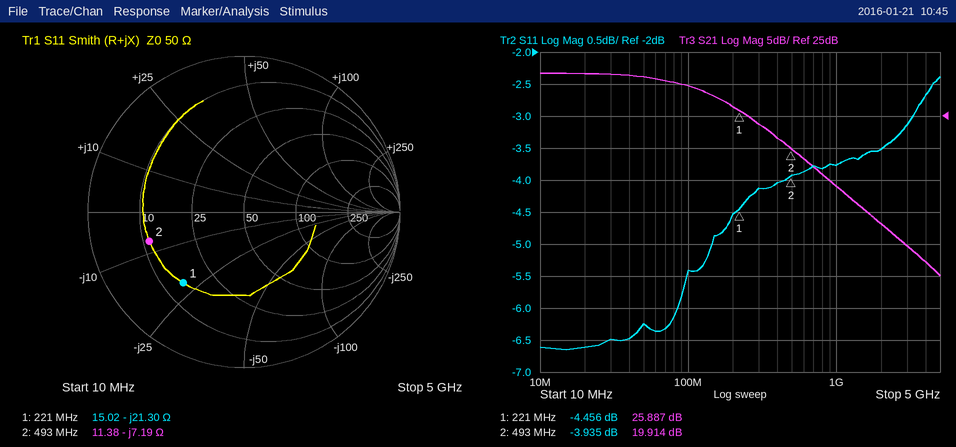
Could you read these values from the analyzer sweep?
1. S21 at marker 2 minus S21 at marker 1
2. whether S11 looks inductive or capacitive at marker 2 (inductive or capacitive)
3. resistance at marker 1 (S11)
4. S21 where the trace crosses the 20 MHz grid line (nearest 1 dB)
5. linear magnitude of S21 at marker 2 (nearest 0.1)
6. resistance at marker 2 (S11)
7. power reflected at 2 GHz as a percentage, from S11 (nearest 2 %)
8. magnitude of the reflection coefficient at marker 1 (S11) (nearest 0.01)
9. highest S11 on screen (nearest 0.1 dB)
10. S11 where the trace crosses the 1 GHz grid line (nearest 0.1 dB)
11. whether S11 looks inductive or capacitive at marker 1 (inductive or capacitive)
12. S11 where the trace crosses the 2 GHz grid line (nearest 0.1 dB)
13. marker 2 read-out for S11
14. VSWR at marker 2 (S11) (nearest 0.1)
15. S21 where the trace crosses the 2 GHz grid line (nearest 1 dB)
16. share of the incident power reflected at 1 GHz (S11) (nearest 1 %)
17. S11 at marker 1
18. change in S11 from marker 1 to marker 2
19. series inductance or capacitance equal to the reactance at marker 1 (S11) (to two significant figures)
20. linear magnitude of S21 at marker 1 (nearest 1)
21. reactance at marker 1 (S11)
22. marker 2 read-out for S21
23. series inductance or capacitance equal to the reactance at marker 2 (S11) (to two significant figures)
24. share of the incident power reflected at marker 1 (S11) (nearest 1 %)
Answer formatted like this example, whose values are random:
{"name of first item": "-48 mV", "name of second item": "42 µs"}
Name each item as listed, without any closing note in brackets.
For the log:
{"S21 at marker 2 minus S21 at marker 1": "-5.973 dB", "whether S11 looks inductive or capacitive at marker 2": "capacitive", "resistance at marker 1": "15.02 Ω", "S21 where the trace crosses the 20 MHz grid line": "32 dB", "linear magnitude of S21 at marker 2": "9.9", "resistance at marker 2": "11.38 Ω", "power reflected at 2 GHz as a percentage, from S11": "44 %", "magnitude of the reflection coefficient at marker 1 (S11)": "0.60", "highest S11 on screen": "-2.4 dB", "S11 where the trace crosses the 1 GHz grid line": "-3.8 dB", "whether S11 looks inductive or capacitive at marker 1": "capacitive", "S11 where the trace crosses the 2 GHz grid line": "-3.5 dB", "marker 2 read-out for S11": "-3.935 dB", "VSWR at marker 2 (S11)": "4.5", "S21 where the trace crosses the 2 GHz grid line": "8 dB", "share of the incident power reflected at 1 GHz (S11)": "42 %", "S11 at marker 1": "-4.456 dB", "change in S11 from marker 1 to marker 2": "0.521 dB", "series inductance or capacitance equal to the reactance at marker 1 (S11)": "34 pF", "linear magnitude of S21 at marker 1": "20", "reactance at marker 1": "-21.30 Ω", "marker 2 read-out for S21": "19.914 dB", "series inductance or capacitance equal to the reactance at marker 2 (S11)": "45 pF", "share of the incident power reflected at marker 1 (S11)": "36 %"}
